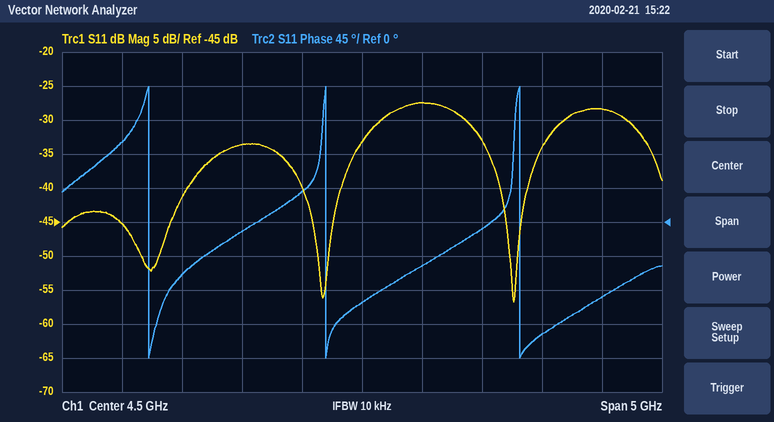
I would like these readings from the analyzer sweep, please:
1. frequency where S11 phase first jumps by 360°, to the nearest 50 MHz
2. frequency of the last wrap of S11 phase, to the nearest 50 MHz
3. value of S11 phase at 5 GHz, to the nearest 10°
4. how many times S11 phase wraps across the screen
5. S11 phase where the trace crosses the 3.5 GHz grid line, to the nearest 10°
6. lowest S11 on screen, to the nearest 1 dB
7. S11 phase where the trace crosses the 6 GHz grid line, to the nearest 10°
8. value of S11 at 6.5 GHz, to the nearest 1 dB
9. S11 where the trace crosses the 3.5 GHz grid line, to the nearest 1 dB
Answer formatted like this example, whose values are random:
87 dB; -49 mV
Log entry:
2.70 GHz; 5.80 GHz; -60°; 3; -10°; -57 dB; -150°; -28 dB; -34 dB
